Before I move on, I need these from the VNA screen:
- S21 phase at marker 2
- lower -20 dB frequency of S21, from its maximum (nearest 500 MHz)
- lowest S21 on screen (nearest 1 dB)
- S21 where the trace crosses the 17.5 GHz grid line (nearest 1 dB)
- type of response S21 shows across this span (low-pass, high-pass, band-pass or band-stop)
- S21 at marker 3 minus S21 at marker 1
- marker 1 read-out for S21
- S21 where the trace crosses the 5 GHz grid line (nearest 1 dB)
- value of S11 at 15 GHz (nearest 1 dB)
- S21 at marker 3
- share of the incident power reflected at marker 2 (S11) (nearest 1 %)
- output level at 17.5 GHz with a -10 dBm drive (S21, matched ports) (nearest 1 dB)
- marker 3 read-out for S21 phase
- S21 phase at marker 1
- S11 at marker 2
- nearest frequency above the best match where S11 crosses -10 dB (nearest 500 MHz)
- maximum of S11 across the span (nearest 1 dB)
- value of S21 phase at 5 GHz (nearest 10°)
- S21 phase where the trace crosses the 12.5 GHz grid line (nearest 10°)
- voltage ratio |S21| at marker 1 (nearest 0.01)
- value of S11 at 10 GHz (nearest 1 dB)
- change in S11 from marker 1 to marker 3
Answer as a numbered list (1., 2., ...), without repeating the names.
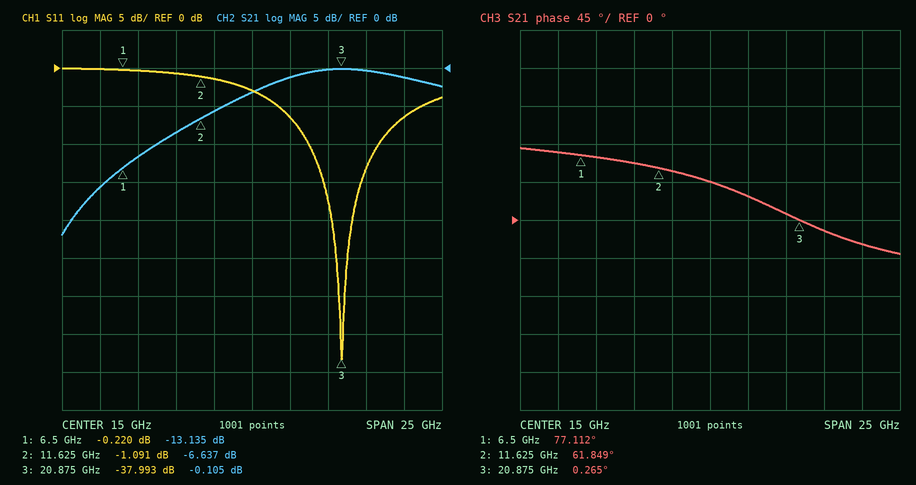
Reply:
1. 61.849°
2. 3.0 GHz
3. -22 dB
4. -1 dB
5. high-pass
6. 13.030 dB
7. -13.135 dB
8. -16 dB
9. -3 dB
10. -0.105 dB
11. 78 %
12. -11 dBm
13. 0.265°
14. 77.112°
15. -1.091 dB
16. 23.5 GHz
17. 0 dB
18. 80°
19. 60°
20. 0.22
21. -1 dB
22. -37.773 dB
